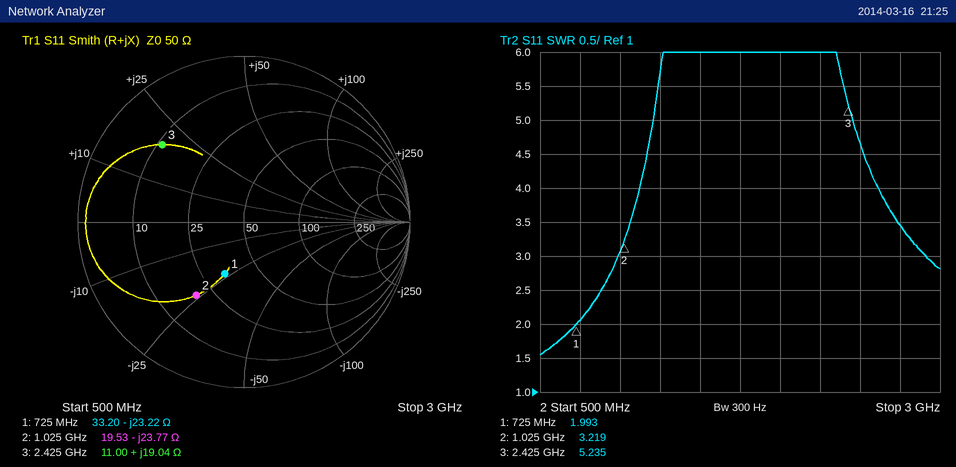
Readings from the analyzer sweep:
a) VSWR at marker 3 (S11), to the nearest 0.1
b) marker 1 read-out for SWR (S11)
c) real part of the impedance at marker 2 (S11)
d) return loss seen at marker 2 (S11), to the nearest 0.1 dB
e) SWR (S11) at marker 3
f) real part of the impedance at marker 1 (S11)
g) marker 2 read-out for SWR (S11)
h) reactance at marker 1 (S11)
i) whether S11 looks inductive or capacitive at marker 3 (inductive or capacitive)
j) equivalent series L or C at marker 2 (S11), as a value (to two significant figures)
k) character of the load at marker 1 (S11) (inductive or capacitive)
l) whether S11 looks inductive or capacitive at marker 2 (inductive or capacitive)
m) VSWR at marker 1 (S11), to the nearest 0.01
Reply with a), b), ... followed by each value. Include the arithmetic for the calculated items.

a) 5.2
b) 1.993
c) 19.53 Ω
d) 5.6 dB
e) 5.235
f) 33.20 Ω
g) 3.219
h) -23.22 Ω
i) inductive
j) C = 1/(2π × 1.025 GHz × 23.77 Ω) ≈ 6.5 pF
k) capacitive
l) capacitive
m) 1.99
